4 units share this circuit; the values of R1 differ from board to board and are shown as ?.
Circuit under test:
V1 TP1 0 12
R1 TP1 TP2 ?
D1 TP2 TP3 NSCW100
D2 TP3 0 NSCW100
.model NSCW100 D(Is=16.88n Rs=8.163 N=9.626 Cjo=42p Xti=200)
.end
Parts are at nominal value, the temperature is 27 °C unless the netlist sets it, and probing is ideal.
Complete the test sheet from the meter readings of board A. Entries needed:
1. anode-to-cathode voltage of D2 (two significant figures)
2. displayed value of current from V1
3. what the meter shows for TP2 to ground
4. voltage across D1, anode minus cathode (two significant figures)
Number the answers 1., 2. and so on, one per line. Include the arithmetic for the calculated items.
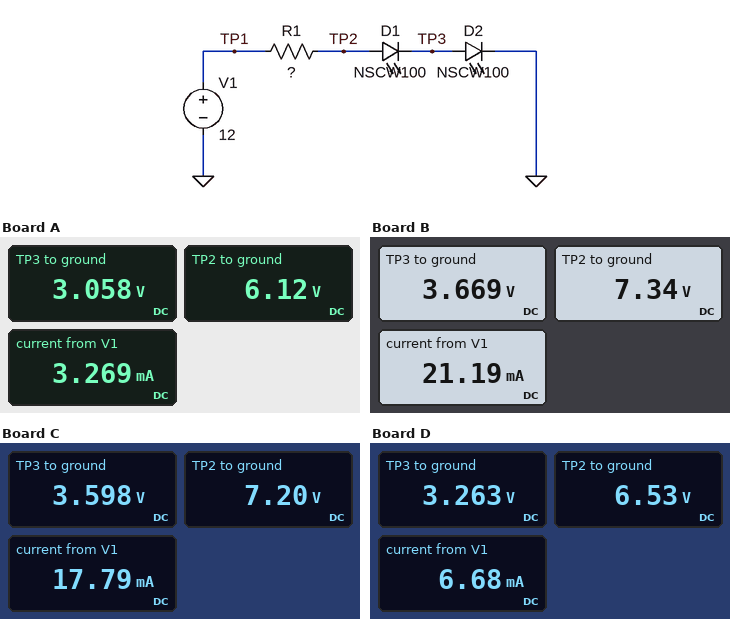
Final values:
1. 3.058 V = 3.1 V
2. 3.269 mA
3. 6.12 V
4. 6.12 V - 3.058 V = 3.1 V
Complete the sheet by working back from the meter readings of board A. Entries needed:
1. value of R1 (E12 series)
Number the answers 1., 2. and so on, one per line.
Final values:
1. 1.8 kΩ
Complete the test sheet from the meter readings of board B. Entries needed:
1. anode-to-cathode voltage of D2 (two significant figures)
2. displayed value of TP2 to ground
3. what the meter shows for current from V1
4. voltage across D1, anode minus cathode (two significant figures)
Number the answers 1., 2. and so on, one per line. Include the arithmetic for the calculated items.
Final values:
1. 3.669 V = 3.7 V
2. 7.34 V
3. 21.19 mA
4. 7.34 V - 3.669 V = 3.7 V
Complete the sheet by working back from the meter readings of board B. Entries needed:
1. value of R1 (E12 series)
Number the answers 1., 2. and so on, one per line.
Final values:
1. 220 Ω
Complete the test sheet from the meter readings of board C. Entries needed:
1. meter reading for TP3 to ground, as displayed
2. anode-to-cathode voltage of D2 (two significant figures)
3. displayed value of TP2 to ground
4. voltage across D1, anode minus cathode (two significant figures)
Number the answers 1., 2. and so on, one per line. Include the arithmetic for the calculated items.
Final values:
1. 3.598 V
2. 3.598 V = 3.6 V
3. 7.20 V
4. 7.2 V - 3.598 V = 3.6 V
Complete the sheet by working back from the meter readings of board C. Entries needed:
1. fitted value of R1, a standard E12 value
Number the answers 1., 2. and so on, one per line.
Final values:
1. 270 Ω
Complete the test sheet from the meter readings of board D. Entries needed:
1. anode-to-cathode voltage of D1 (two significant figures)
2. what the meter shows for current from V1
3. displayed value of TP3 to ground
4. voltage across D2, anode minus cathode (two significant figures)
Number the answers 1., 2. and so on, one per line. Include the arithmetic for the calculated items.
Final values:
1. 6.53 V - 3.263 V = 3.3 V
2. 6.68 mA
3. 3.263 V
4. 3.263 V = 3.3 V
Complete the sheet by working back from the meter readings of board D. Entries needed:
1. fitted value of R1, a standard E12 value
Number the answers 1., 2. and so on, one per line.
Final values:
1. 820 Ω
